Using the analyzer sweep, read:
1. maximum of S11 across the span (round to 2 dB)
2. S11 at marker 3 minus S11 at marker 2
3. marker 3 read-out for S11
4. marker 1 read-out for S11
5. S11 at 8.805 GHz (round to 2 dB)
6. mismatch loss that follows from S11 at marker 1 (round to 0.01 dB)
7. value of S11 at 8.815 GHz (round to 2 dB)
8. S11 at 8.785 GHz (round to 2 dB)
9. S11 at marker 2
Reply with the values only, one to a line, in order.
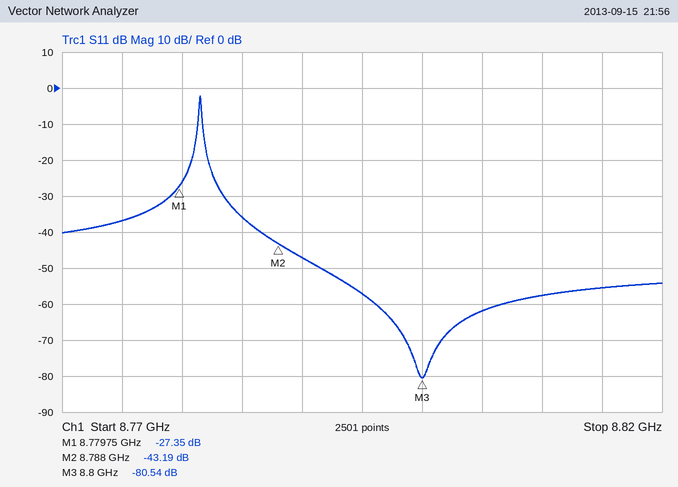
-2 dB
-37.35 dB
-80.54 dB
-27.35 dB
-62 dB
0.01 dB
-56 dB
-36 dB
-43.19 dB
